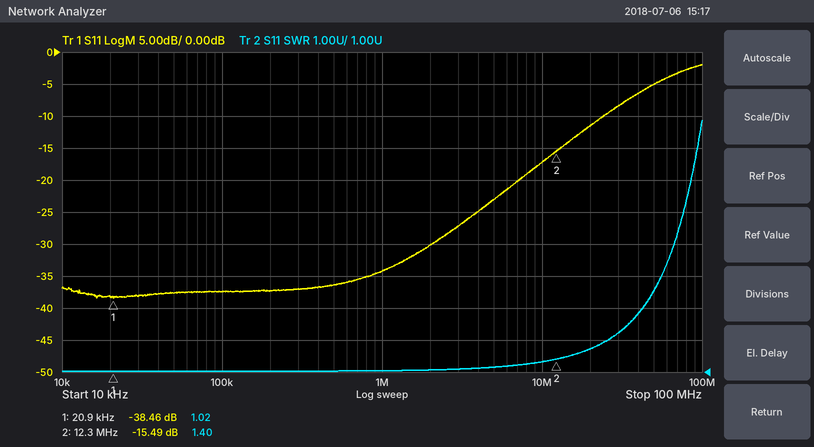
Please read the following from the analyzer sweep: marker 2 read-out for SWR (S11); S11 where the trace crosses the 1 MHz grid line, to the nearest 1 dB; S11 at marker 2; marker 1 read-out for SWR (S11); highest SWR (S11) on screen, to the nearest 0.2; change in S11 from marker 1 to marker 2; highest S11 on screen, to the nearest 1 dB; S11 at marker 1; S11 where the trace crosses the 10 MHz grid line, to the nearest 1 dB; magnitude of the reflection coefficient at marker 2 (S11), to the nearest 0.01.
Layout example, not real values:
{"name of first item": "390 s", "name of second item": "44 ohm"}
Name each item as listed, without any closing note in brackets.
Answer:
{"marker 2 read-out for SWR": "1.40", "S11 where the trace crosses the 1 MHz grid line, to the nearest 1 dB": "-34 dB", "S11 at marker 2": "-15.49 dB", "marker 1 read-out for SWR": "1.02", "highest SWR (S11) on screen, to the nearest 0.2": "8.8", "change in S11 from marker 1 to marker 2": "22.97 dB", "highest S11 on screen, to the nearest 1 dB": "-2 dB", "S11 at marker 1": "-38.46 dB", "S11 where the trace crosses the 10 MHz grid line, to the nearest 1 dB": "-17 dB", "magnitude of the reflection coefficient at marker 2 (S11), to the nearest 0.01": "0.17"}
